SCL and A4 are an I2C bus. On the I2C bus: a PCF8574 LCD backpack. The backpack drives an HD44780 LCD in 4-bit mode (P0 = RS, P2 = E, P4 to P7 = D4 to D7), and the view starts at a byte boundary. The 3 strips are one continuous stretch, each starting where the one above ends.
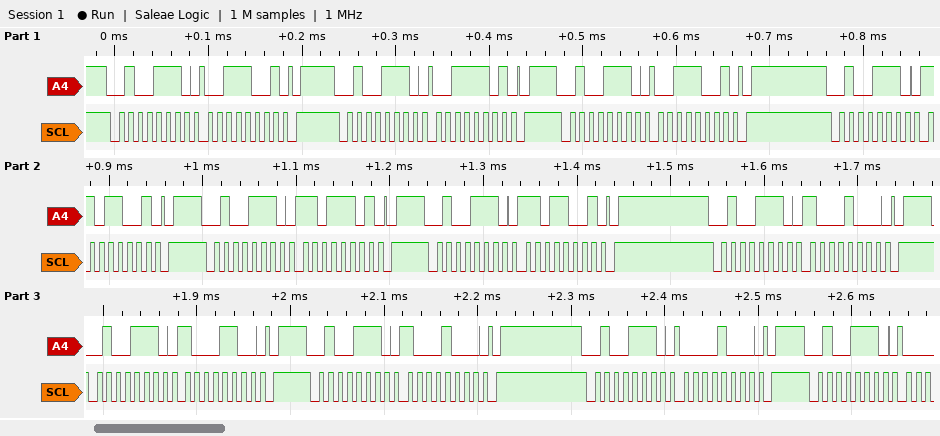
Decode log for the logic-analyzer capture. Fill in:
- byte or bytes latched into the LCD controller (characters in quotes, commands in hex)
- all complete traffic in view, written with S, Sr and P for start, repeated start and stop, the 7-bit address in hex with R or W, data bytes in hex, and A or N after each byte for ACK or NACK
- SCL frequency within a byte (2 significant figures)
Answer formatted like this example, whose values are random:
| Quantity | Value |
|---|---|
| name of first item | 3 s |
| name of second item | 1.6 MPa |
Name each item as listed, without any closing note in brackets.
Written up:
| Quantity | Value |
|---|---|
| byte or bytes latched into the LCD controller | '=' |
| all complete traffic in view, written with S, Sr and P for start, repeated start and stop, the 7-bit address in hex with R or W, data bytes in hex, and A or N after each byte for ACK or NACK | S 27W A 39 A P S 27W A 3D A P S 27W A 39 A P S 27W A D9 A P S 27W A DD A P S 27W A D9 A P S 27W A 88 A P S 27W A 8C A P S 27W A 88 A P S 27W A 08 A P S 27W A |
| SCL frequency within a byte | 100 kHz |
